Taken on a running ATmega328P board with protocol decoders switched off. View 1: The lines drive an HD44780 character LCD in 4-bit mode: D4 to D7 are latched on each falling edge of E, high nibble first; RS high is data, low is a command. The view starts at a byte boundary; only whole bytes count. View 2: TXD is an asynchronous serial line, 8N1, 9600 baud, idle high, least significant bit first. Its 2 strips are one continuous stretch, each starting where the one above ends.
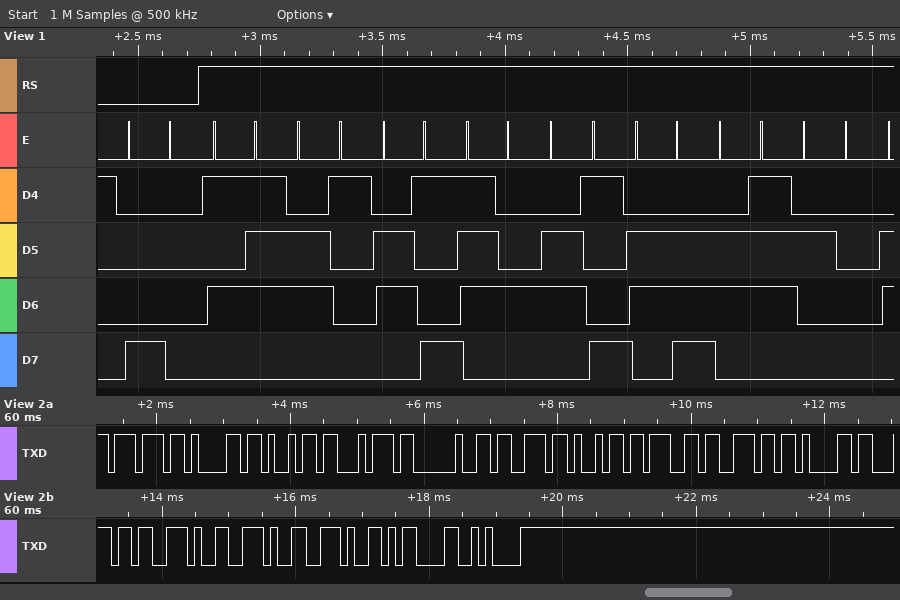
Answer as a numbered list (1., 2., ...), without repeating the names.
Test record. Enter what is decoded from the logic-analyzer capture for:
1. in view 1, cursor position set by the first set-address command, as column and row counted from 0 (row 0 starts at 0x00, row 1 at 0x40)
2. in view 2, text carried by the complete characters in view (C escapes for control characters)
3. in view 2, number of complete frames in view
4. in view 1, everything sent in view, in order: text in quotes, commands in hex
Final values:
1. column 0, row 0
2. "wait signal...\r\n"
3. 16
4. 0x80 "Waiting "
